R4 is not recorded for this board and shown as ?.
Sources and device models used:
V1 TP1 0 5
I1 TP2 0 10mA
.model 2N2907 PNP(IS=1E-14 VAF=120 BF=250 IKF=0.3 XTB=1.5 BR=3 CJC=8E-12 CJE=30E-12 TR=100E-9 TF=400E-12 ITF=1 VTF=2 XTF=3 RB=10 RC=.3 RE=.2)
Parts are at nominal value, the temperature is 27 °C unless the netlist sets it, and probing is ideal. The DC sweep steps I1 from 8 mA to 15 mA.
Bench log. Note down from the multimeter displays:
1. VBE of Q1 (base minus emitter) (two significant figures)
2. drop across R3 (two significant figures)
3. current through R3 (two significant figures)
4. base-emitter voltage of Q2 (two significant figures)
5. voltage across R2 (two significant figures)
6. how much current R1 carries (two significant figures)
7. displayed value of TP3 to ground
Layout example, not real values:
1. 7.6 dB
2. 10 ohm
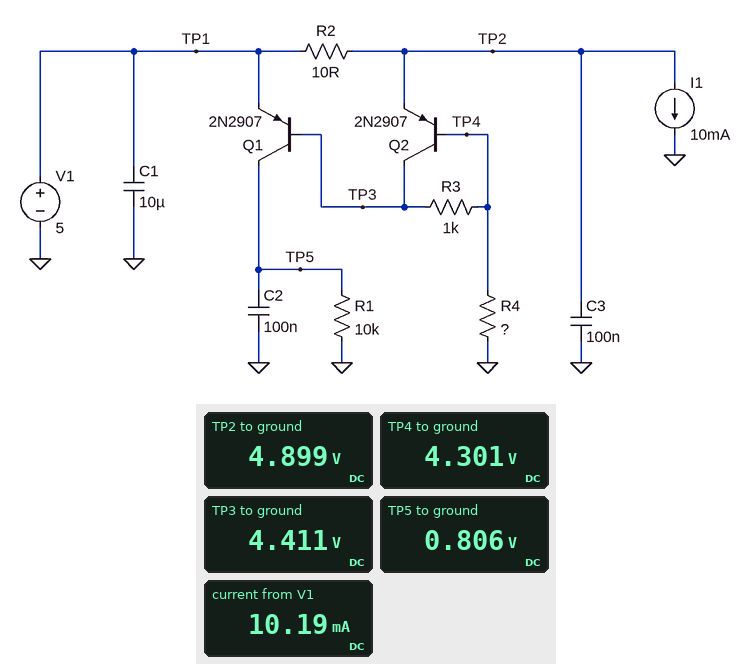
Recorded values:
1. -590 mV
2. 110 mV
3. 110 µA
4. -600 mV
5. 100 mV
6. 81 µA
7. 4.411 V
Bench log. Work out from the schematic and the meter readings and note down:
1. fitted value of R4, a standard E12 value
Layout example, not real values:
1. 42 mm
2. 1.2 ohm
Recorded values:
1. 39 kΩ
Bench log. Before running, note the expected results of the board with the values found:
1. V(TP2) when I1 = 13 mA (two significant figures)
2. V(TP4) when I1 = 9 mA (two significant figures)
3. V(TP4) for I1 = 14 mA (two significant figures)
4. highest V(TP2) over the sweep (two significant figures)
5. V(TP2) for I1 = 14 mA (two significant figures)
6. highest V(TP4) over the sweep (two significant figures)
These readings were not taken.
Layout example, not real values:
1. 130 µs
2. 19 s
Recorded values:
1. 4.9 V
2. 4.3 V
3. 4.3 V
4. 4.9 V
5. 4.9 V
6. 4.3 V
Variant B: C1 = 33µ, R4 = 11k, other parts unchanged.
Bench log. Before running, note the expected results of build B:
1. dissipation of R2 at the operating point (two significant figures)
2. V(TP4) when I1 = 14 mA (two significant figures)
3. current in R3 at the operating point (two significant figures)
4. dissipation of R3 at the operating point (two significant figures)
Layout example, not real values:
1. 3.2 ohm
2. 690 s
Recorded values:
1. 1.1 mW
2. 4.2 V
3. 390 µA
4. 150 µW
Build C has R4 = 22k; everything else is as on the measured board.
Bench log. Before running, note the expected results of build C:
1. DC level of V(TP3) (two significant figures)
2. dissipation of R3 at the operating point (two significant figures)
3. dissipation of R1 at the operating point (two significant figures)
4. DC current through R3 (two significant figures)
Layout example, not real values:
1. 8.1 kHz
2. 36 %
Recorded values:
1. 4.5 V
2. 38 µW
3. 330 nW
4. 190 µA
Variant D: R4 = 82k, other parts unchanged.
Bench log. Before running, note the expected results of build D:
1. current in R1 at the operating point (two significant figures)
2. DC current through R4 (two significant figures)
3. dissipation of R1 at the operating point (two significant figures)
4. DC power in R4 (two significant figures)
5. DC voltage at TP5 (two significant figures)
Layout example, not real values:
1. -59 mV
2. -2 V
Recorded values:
1. 330 µA
2. 53 µA
3. 1.1 mW
4. 230 µW
5. 3.3 V
